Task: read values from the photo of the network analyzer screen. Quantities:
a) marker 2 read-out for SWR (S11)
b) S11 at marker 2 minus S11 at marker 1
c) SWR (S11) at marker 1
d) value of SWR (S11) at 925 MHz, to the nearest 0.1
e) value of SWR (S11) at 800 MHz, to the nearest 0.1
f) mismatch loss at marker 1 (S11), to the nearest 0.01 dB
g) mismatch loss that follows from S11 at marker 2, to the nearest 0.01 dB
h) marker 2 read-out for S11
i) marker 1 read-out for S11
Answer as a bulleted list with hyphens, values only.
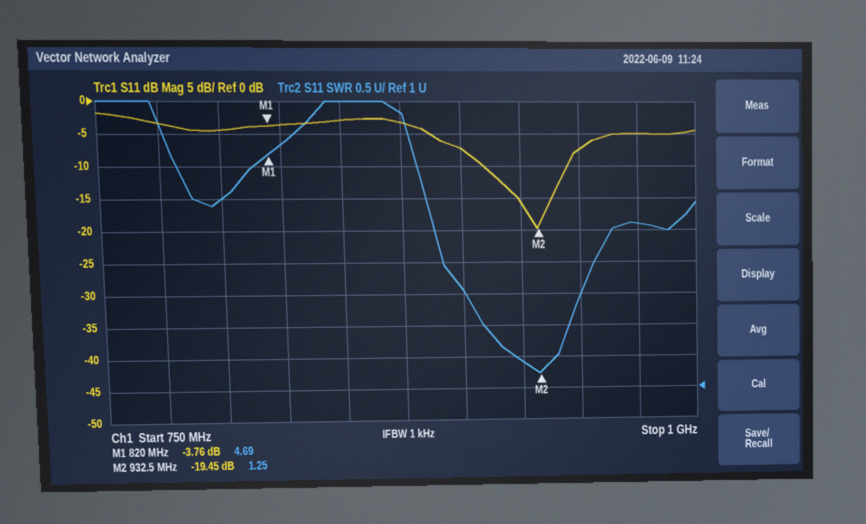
- 1.25
- -15.69 dB
- 4.69
- 1.4
- 4.0
- 2.37 dB
- 0.05 dB
- -19.45 dB
- -3.76 dB
